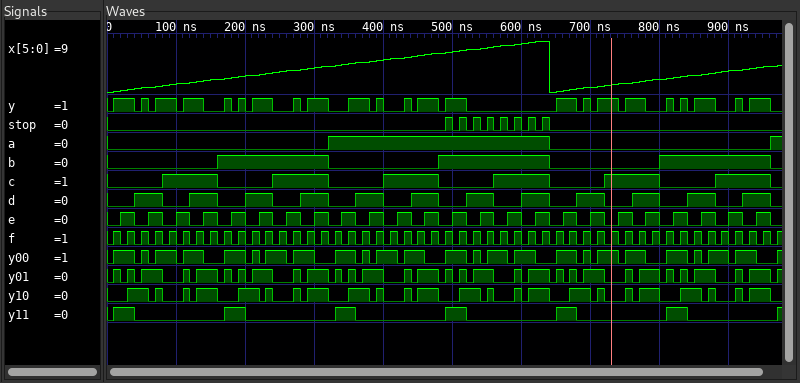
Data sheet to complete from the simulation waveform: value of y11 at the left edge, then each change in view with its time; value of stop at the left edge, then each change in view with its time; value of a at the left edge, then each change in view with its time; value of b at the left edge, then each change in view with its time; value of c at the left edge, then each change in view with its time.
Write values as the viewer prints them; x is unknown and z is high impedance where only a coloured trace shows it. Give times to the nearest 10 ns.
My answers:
0, 1 at 10 ns, 0 at 40 ns, 1 at 170 ns, 0 at 200 ns, 1 at 330 ns, 0 at 360 ns, 1 at 490 ns, 0 at 520 ns, 1 at 650 ns, 0 at 680 ns, 1 at 810 ns, 0 at 840 ns, 1 at 970 ns
0, 1 at 490 ns, 0 at 500 ns, 1 at 510 ns, 0 at 520 ns, 1 at 530 ns, 0 at 540 ns, 1 at 550 ns, 0 at 560 ns, 1 at 570 ns, 0 at 580 ns, 1 at 590 ns, 0 at 600 ns, 1 at 610 ns, 0 at 620 ns, 1 at 630 ns, 0 at 640 ns
0, 1 at 320 ns, 0 at 640 ns, 1 at 960 ns
0, 1 at 160 ns, 0 at 320 ns, 1 at 480 ns, 0 at 640 ns, 1 at 800 ns, 0 at 960 ns
0, 1 at 80 ns, 0 at 160 ns, 1 at 240 ns, 0 at 320 ns, 1 at 400 ns, 0 at 480 ns, 1 at 560 ns, 0 at 640 ns, 1 at 720 ns, 0 at 800 ns, 1 at 880 ns, 0 at 960 ns
